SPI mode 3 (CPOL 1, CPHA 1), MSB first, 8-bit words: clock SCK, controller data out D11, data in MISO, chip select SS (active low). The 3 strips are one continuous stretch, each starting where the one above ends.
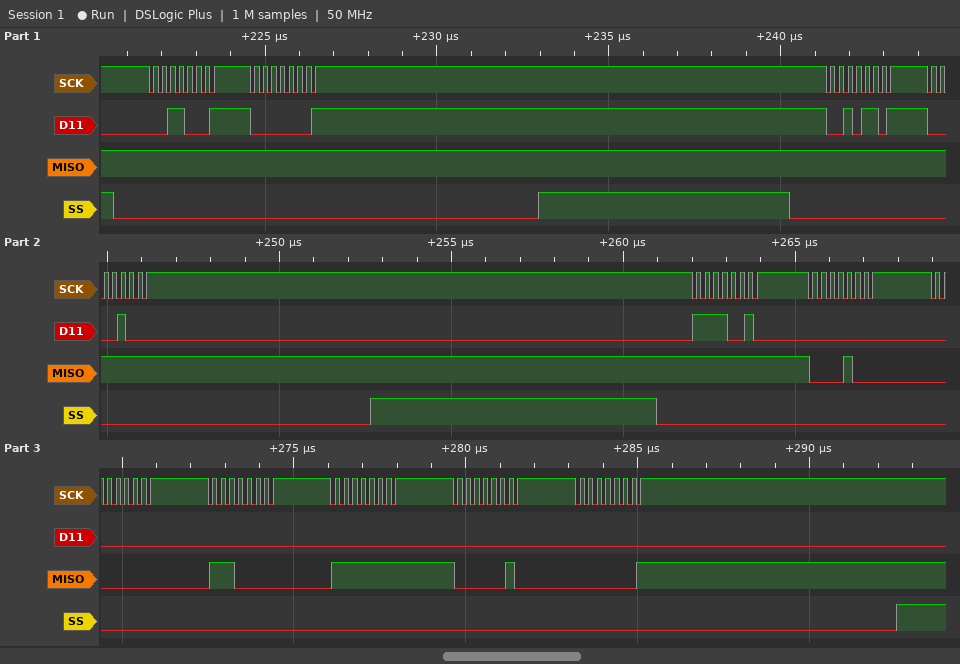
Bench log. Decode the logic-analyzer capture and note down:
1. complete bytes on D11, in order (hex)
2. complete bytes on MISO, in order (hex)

31 01 2D 08 F2 00 00 00 00 00 00
FF FF FF FF FF 08 00 E0 FF 02 01
